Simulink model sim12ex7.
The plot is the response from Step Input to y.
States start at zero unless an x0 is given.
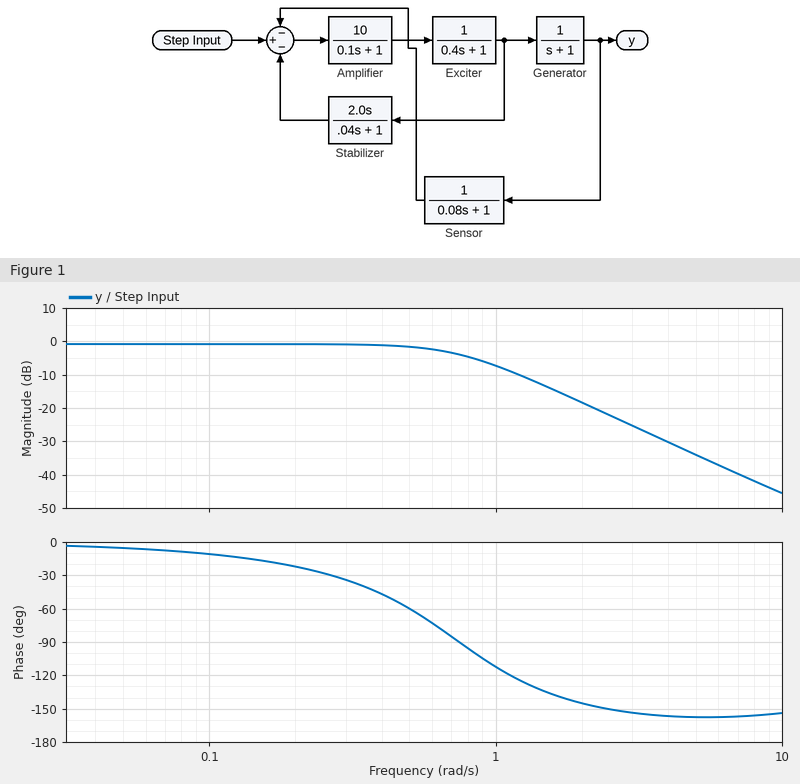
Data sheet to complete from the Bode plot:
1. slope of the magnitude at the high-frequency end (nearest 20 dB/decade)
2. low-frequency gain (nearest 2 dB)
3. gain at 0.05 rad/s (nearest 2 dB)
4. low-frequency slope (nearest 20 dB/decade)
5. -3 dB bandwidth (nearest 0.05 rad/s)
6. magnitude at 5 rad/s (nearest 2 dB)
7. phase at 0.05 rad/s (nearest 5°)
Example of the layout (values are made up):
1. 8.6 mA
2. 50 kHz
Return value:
1. -40 dB/decade
2. 0 dB
3. 0 dB
4. 0 dB/decade
5. 0.75 rad/s
6. -34 dB
7. -5°
